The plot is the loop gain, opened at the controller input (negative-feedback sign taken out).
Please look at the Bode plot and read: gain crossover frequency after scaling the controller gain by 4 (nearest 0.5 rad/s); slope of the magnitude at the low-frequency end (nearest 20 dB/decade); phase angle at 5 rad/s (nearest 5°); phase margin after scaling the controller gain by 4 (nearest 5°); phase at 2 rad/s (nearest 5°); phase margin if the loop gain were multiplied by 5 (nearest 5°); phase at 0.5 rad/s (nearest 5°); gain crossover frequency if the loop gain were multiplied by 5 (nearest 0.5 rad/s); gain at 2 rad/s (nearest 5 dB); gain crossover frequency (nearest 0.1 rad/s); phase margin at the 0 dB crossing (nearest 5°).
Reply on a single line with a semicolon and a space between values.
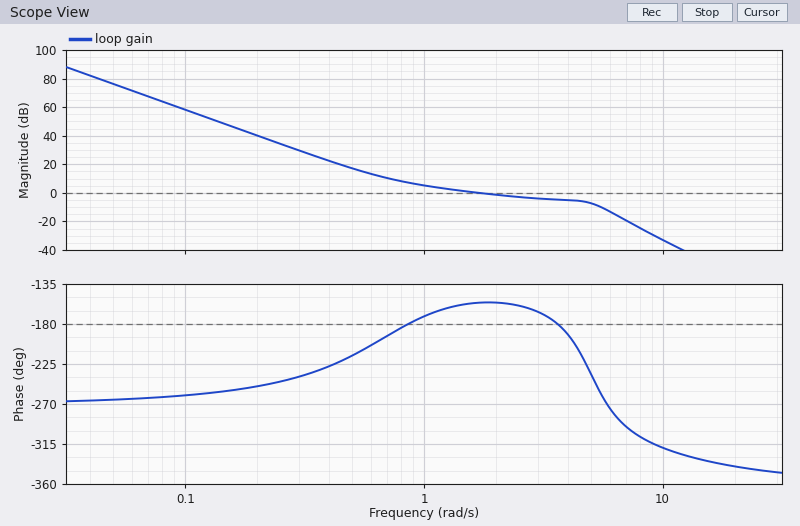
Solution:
6.0 rad/s; -60 dB/decade; -235°; -90°; -155°; -100°; -215°; 6.0 rad/s; 0 dB; 1.7 rad/s; 25°
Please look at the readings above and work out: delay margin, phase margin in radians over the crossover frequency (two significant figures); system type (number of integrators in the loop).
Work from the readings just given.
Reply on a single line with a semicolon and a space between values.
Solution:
0.26 s; 3
